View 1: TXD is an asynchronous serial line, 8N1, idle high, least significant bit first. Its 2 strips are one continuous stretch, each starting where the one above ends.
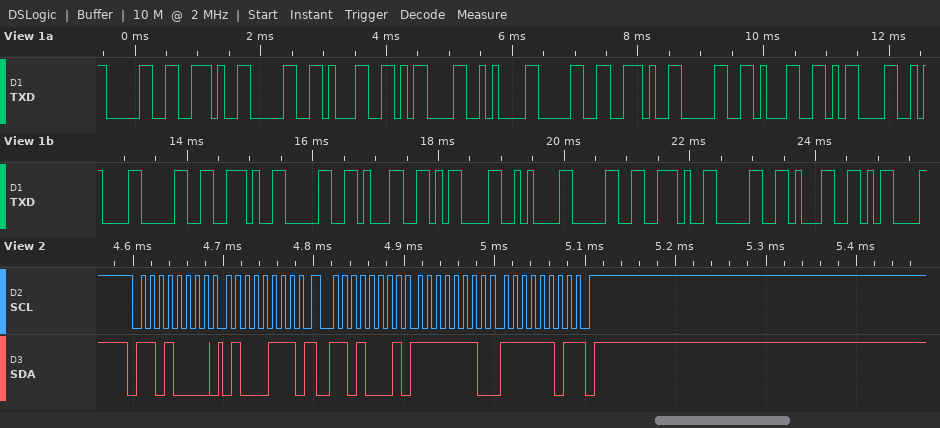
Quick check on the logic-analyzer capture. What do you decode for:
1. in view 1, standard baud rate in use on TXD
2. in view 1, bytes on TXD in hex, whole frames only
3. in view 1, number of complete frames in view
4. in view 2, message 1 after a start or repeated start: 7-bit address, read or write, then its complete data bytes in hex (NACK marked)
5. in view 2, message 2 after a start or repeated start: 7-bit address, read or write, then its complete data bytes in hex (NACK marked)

9600 baud
30 2E 30 31 0D 0A 30 2E 30 31 0D 0A 30 2E 30 31 0D 0A 30 2E 30 31 0D
23
0x68 write: 47
0x68 read: FE FD NACK
